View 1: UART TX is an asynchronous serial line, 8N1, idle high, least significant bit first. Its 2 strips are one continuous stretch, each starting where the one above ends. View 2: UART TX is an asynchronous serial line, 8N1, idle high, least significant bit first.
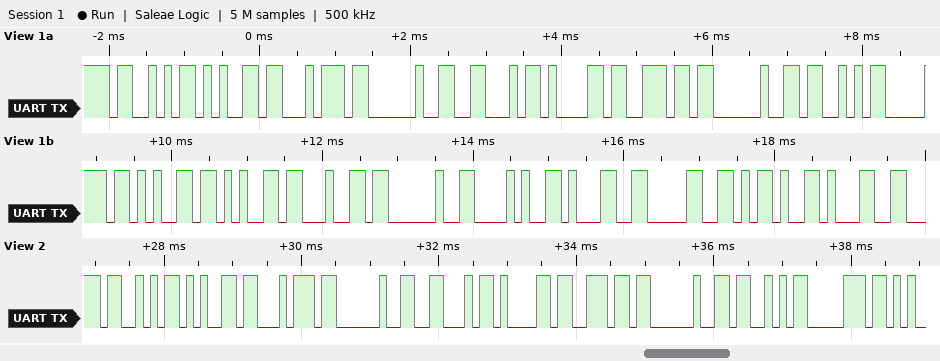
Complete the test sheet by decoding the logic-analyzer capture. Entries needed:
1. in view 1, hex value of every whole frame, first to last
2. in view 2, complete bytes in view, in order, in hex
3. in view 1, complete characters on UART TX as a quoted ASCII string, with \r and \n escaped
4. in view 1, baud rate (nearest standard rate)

53 65 74 20 46 61 6E 20 53 70 65 65 64 20 28 31 30 2D 31
53 65 74 20 46 61 6E 20 53 70
"Set Fan Speed (10-1"
9600 baud
